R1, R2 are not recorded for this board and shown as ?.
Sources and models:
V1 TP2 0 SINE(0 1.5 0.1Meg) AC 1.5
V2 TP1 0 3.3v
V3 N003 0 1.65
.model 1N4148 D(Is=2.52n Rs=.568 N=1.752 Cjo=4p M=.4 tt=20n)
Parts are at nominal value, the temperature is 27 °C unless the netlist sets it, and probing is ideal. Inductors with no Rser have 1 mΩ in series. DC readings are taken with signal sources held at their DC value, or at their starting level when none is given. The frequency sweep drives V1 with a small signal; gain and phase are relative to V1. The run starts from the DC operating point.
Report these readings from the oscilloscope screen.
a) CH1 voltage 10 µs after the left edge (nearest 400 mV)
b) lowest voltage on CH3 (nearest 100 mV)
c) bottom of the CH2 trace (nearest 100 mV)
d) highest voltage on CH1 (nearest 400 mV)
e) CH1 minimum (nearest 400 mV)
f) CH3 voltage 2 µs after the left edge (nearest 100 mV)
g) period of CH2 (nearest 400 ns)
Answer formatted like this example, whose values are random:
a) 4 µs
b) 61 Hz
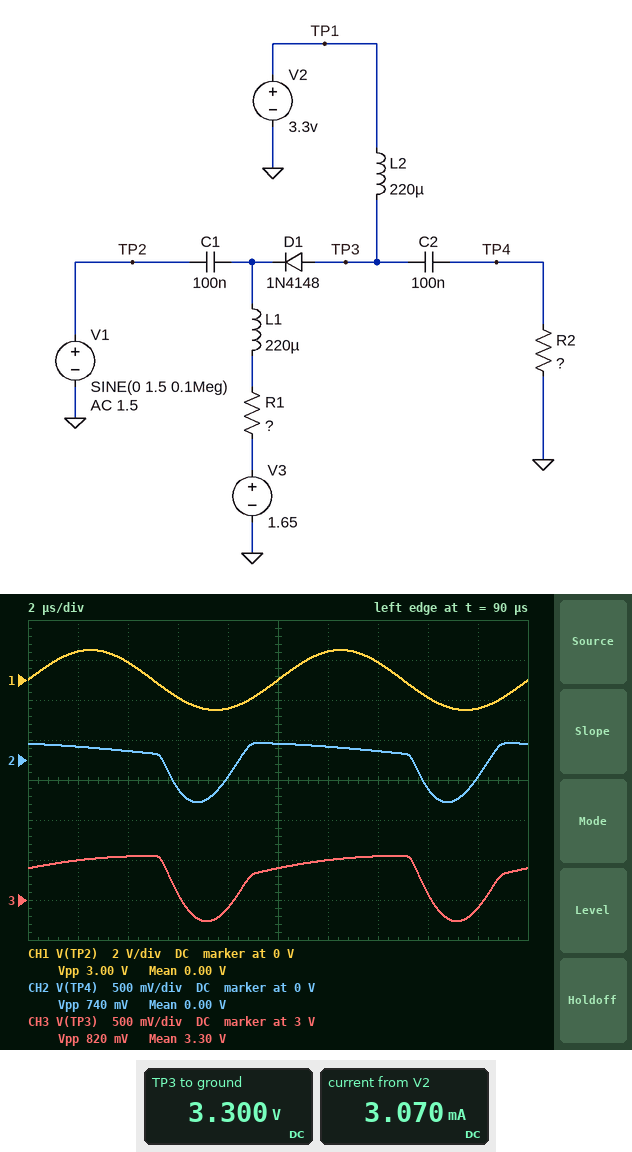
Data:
a) 0 V
b) 2.7 V
c) -500 mV
d) 1.6 V
e) -1.6 V
f) 3.5 V
g) 10.0 µs
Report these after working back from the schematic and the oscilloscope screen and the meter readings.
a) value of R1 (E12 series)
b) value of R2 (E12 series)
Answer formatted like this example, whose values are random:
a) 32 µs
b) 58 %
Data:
a) 330 Ω
b) 27 Ω
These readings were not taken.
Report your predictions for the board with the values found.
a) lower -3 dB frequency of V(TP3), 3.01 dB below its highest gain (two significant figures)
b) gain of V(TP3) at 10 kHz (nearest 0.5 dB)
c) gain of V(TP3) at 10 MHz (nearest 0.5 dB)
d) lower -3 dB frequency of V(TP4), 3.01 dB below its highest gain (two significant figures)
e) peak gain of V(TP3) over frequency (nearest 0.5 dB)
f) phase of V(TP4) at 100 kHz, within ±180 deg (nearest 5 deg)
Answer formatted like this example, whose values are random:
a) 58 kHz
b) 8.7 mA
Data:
a) 21 kHz
b) -20.0 dB
c) -2.0 dB
d) 4.8 MHz
e) 2.0 dB
f) 45 deg
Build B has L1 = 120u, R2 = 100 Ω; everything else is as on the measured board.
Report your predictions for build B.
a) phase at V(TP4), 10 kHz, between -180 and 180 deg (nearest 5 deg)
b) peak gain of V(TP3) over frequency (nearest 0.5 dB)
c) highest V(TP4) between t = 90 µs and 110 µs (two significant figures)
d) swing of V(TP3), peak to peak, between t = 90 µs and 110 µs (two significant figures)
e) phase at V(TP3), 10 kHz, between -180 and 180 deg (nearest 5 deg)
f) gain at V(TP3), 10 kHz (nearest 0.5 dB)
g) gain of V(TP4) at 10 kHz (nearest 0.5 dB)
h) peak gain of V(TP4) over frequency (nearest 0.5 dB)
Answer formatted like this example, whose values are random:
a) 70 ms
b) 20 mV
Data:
a) -135 deg
b) 1.5 dB
c) 850 mV
d) 1.7 V
e) 170 deg
f) -20.5 dB
g) -26.0 dB
h) 0.5 dB
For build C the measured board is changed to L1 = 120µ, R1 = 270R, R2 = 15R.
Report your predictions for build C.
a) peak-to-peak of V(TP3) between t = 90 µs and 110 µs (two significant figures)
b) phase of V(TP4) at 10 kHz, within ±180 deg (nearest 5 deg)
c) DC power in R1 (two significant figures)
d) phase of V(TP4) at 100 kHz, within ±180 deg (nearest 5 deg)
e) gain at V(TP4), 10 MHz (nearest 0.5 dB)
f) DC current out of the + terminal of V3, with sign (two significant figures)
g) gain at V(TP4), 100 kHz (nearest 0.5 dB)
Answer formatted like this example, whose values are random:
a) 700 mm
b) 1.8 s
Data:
a) 760 mV
b) -105 deg
c) 3.7 mW
d) 55 deg
e) -3.0 dB
f) -3.7 mA
g) -8.5 dB
